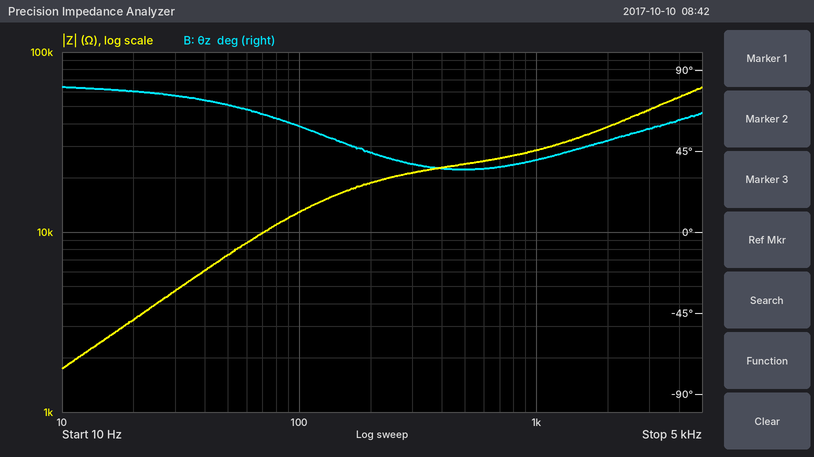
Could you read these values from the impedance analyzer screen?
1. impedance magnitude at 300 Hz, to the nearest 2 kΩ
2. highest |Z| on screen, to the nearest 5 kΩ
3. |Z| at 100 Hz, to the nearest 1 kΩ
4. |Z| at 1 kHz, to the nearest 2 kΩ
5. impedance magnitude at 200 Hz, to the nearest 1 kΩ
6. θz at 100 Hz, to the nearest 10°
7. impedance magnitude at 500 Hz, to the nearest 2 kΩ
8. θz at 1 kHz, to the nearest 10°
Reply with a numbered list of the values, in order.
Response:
1. 22 kΩ
2. 65 kΩ
3. 13 kΩ
4. 28 kΩ
5. 19 kΩ
6. 60°
7. 24 kΩ
8. 40°
